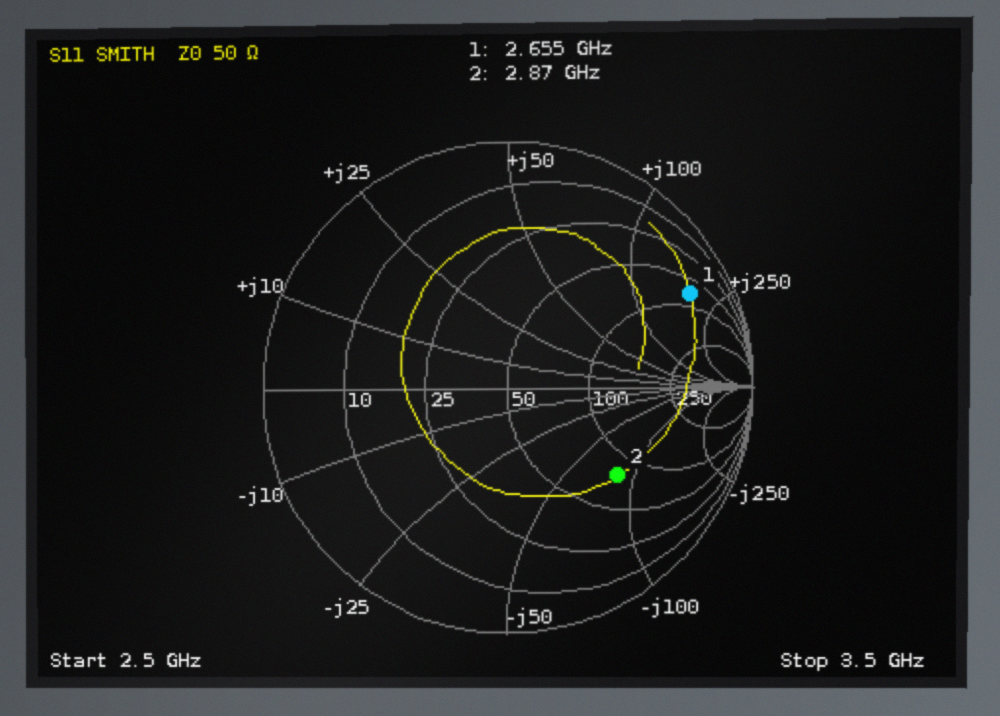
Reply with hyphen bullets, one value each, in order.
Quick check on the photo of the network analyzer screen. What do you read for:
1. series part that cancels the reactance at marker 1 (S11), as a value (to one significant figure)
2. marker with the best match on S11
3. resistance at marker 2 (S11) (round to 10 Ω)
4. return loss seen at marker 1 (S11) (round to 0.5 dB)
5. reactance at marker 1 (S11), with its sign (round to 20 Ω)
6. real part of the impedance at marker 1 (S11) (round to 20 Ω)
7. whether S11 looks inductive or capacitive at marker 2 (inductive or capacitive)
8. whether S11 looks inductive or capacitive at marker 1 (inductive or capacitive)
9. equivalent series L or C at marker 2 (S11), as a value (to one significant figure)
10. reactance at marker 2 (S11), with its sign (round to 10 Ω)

- 300 fF
- marker 2
- 80 Ω
- 1.5 dB
- +180 Ω
- 80 Ω
- capacitive
- inductive
- 700 fF
- -80 Ω
